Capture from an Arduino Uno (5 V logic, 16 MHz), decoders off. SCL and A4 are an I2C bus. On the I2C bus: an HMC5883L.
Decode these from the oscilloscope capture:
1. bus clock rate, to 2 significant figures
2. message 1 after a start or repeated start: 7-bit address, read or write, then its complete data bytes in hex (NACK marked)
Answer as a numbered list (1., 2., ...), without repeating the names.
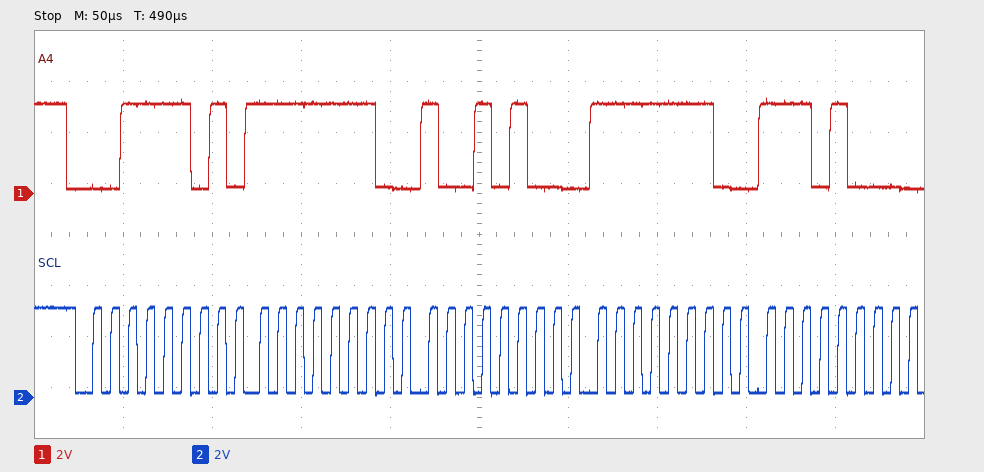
1. 100 kHz
2. 0x1E read: FE 94 FE E8
